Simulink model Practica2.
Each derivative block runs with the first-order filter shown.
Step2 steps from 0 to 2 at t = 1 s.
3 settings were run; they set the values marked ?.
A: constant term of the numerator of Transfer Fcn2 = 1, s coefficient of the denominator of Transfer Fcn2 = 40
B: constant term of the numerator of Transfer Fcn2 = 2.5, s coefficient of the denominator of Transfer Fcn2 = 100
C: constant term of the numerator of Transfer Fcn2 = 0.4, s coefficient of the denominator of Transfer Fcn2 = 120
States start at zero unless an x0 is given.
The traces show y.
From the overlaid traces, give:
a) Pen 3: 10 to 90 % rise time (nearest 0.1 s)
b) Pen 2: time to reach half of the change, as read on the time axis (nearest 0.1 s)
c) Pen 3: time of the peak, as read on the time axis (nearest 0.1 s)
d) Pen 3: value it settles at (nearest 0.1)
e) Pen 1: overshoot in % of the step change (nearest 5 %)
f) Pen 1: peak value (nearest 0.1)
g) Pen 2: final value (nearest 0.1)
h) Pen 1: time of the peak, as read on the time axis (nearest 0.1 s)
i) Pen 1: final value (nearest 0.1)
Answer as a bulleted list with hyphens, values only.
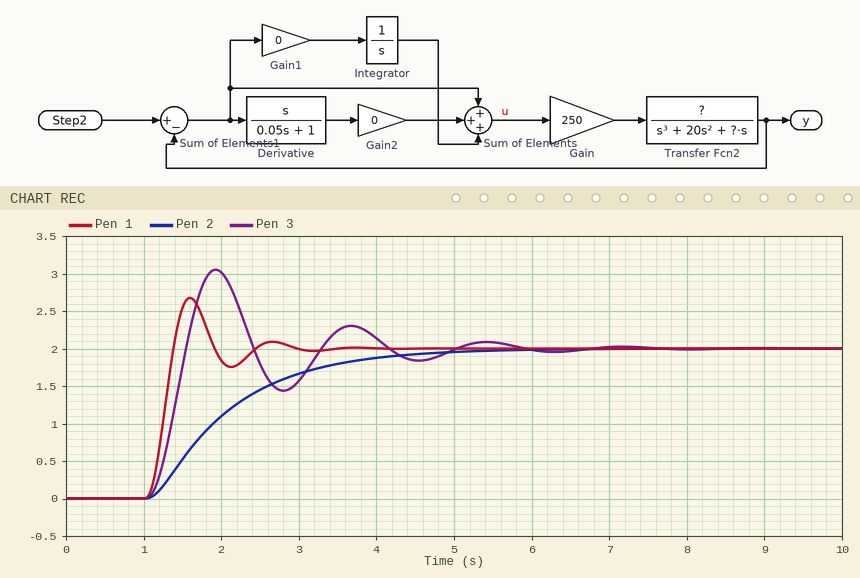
- 0.3 s
- 1.9 s
- 1.9 s
- 2.0
- 35 %
- 2.7
- 2.0
- 1.6 s
- 2.0
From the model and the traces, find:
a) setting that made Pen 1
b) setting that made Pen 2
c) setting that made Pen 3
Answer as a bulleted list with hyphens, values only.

- B
- C
- A
